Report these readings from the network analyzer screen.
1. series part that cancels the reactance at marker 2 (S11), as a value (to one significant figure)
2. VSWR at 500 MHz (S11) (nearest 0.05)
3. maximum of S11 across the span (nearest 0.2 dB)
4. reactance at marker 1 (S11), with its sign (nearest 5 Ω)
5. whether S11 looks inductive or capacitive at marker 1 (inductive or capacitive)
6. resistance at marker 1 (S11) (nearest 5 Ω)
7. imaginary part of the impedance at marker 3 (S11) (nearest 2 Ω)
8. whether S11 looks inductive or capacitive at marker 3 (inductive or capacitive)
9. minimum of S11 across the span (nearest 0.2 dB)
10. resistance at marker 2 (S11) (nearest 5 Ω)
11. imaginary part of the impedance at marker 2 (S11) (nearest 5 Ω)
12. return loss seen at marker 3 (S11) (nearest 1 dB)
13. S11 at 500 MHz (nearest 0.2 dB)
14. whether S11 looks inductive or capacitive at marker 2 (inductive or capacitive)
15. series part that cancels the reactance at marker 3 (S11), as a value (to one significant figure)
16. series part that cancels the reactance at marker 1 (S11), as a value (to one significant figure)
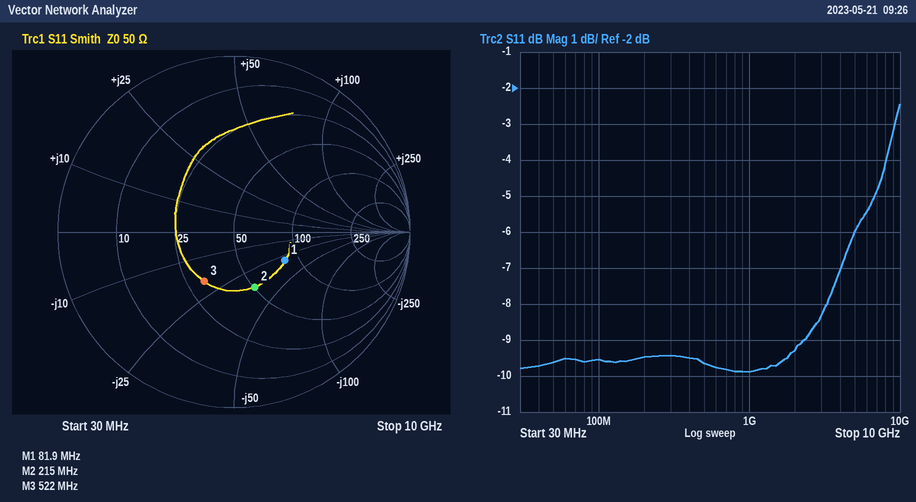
30 nH
2.00
-2.4 dB
-30 Ω
capacitive
85 Ω
-20 Ω
capacitive
-9.8 dB
50 Ω
-35 Ω
10 dB
-9.6 dB
capacitive
6 nH
60 nH
